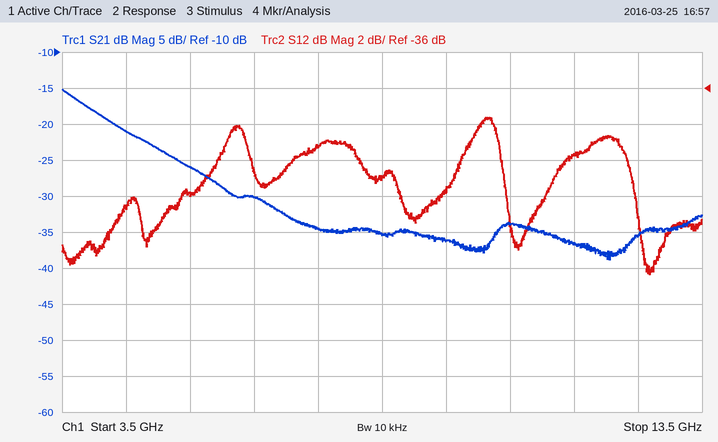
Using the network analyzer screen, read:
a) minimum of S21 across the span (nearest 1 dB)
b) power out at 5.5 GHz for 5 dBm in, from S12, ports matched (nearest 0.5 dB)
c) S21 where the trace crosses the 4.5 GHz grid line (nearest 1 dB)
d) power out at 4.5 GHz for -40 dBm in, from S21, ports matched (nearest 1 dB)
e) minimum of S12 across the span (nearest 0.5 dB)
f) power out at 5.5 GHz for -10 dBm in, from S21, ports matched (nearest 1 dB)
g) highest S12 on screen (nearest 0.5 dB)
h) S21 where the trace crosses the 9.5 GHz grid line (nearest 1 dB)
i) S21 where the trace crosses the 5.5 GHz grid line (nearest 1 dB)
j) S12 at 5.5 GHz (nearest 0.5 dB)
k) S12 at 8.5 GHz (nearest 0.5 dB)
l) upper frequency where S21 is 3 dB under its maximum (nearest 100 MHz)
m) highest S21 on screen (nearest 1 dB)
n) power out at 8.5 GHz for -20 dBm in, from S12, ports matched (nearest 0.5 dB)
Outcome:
-39 dB
-37.0 dBm
-21 dB
-61 dBm
-46.5 dB
-36 dBm
-37.5 dB
-36 dB
-26 dB
-42.0 dB
-41.0 dB
4.0 GHz
-15 dB
-61.0 dBm
